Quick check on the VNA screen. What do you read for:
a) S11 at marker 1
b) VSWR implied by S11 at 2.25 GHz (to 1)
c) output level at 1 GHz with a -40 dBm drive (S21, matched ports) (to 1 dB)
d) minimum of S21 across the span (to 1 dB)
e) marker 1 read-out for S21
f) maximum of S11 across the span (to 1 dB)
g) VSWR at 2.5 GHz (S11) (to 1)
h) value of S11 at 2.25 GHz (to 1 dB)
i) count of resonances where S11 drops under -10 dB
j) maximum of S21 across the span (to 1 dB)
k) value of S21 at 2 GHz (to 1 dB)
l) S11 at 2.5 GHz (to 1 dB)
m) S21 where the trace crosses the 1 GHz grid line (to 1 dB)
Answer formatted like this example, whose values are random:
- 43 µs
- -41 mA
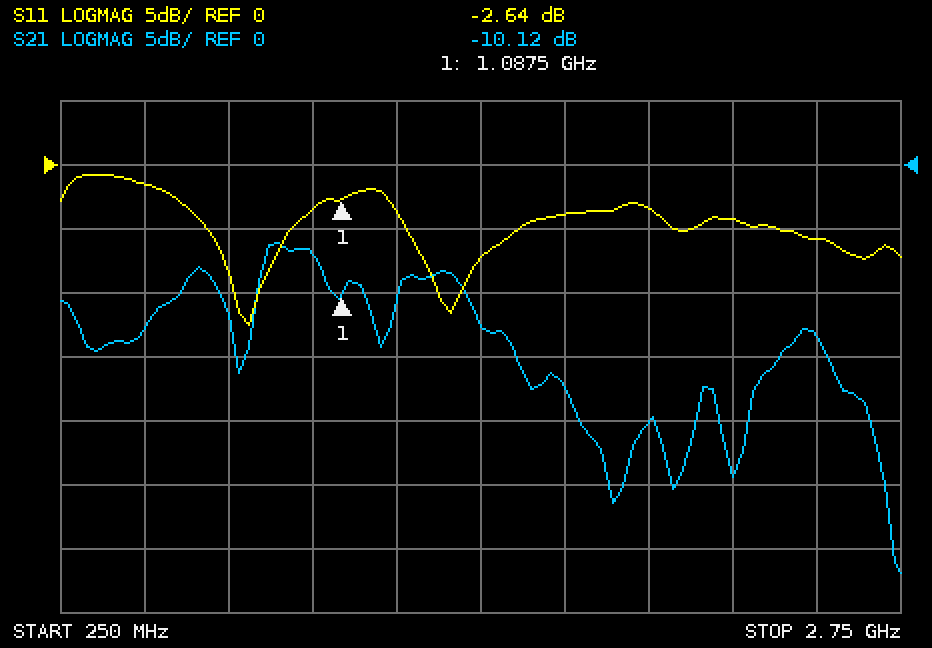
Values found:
- -2.64 dB
- 4
- -47 dBm
- -32 dB
- -10.12 dB
- -1 dB
- 3
- -4 dB
- 2
- -6 dB
- -20 dB
- -6 dB
- -7 dB
